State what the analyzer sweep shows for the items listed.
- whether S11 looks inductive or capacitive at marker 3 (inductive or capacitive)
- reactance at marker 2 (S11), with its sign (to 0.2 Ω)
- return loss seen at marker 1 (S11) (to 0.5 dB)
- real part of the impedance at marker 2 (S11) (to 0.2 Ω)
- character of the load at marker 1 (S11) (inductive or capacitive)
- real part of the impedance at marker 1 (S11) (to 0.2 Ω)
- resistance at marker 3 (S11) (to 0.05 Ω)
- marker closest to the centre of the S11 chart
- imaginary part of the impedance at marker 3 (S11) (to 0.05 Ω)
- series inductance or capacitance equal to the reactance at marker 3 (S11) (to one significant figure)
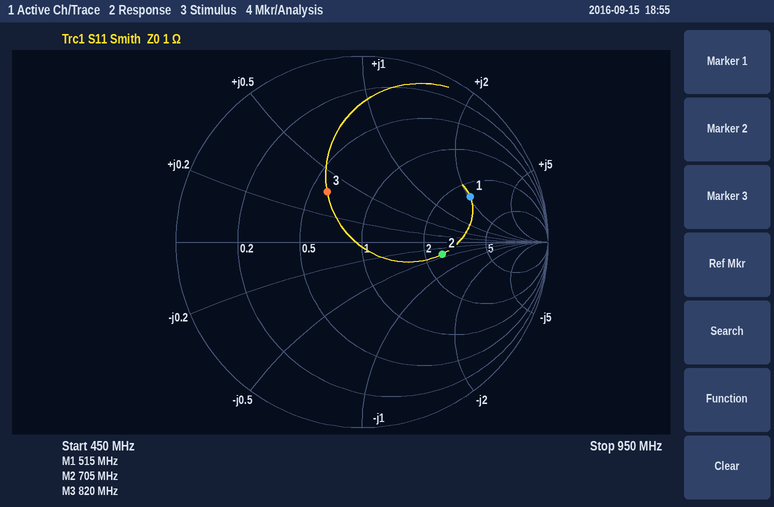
inductive
-0.4 Ω
4.0 dB
2.4 Ω
inductive
2.6 Ω
0.60 Ω
marker 3
+0.35 Ω
70 pH
